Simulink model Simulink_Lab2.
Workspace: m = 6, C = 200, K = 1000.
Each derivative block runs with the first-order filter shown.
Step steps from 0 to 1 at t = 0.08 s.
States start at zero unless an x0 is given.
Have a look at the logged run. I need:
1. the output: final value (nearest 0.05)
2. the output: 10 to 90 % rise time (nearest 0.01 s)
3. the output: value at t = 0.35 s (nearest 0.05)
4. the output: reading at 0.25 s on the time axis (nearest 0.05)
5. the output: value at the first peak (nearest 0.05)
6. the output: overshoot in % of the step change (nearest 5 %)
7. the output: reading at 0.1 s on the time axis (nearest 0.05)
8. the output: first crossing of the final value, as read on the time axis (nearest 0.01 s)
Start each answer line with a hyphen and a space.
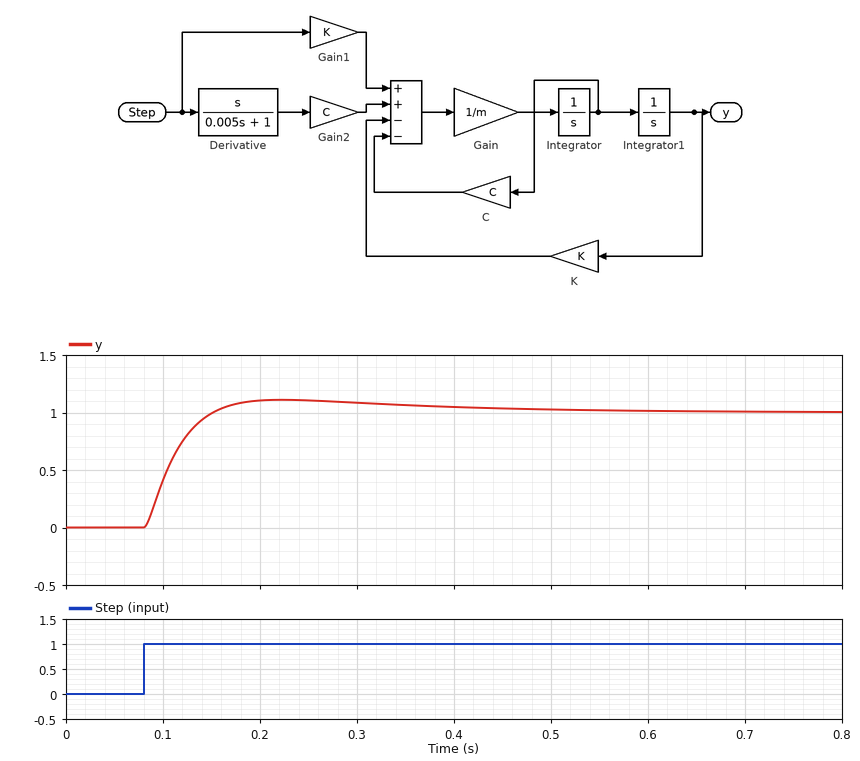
- 1.00
- 0.05 s
- 1.05
- 1.10
- 1.10
- 10 %
- 0.40
- 0.15 s
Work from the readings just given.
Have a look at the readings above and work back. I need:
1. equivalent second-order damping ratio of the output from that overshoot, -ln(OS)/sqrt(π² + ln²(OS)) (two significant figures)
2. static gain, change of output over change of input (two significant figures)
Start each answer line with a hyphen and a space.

- 0.59
- 1.0
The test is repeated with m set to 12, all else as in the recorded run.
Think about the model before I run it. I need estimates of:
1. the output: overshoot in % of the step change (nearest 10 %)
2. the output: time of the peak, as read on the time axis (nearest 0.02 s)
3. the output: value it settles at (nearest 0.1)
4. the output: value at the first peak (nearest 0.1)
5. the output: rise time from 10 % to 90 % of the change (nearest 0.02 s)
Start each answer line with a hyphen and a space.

- 20 %
- 0.30 s
- 1.0
- 1.2
- 0.08 s
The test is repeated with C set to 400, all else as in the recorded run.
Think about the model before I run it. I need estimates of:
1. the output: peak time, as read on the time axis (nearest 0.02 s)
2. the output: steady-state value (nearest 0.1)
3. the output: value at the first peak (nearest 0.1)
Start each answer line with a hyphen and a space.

- 0.18 s
- 1.0
- 1.0
